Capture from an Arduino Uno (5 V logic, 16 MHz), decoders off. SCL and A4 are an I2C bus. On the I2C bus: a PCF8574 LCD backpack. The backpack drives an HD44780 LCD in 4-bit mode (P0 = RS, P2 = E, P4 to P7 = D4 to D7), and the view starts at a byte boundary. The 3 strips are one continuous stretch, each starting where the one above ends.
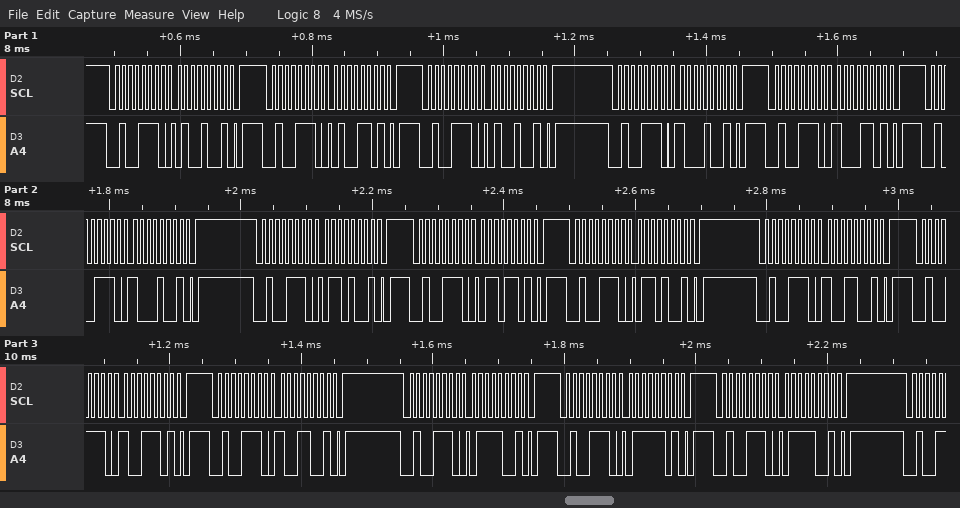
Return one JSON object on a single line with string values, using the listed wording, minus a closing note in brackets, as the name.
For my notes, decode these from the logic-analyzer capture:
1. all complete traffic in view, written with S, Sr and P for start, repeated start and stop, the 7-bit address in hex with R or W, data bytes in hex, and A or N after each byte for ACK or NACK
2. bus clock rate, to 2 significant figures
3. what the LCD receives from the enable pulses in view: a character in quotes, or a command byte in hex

{"all complete traffic in view, written with S, Sr and P for start, repeated start and stop, the 7-bit address in hex with R or W, data bytes in hex, and A or N after each byte for ACK or NACK": "S 27W A 49 A P S 27W A 4D A P S 27W A 49 A P S 27W A 89 A P S 27W A 8D A P S 27W A 89 A P S 27W A 69 A P S 27W A 6D A P S 27W A 69 A P S 27W A 99 A P S 27W A 9D A P S 27W A 99 A P S 27W A 79 A P S 27W A 7D A P S 27W A 79 A P", "bus clock rate, to 2 significant figures": "100 kHz", "what the LCD receives from the enable pulses in view: a character in quotes, or a command byte in hex": "'H' 'i'"}
